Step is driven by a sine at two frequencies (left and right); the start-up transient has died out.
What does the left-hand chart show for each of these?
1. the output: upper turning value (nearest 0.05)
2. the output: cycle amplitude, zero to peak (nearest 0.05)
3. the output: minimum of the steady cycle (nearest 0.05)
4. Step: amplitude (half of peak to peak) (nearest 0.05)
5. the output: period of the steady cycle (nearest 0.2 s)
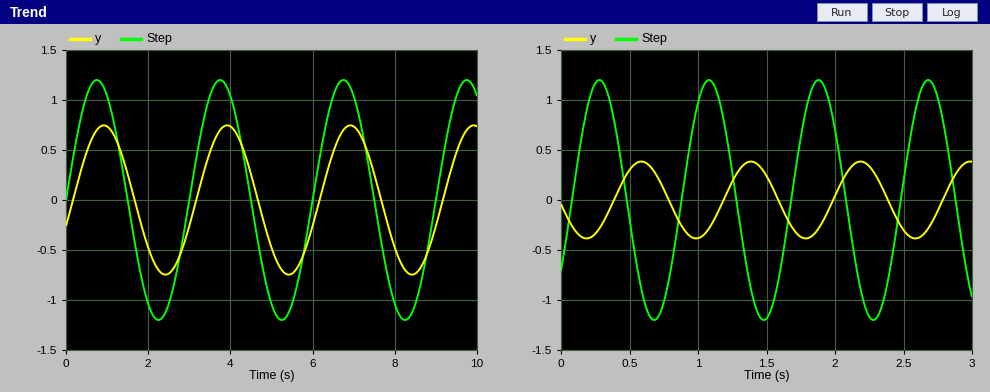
0.75
0.75
-0.75
1.20
3.0 s
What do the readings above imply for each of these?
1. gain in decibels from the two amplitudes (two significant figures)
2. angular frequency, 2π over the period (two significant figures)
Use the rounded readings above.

-4.1 dB
2.1 rad/s
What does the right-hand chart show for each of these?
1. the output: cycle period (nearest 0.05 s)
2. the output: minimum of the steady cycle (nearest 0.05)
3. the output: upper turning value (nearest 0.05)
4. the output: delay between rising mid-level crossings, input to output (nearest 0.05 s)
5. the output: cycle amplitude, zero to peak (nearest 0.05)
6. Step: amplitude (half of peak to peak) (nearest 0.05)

0.80 s
-0.40
0.40
0.30 s
0.40
1.20
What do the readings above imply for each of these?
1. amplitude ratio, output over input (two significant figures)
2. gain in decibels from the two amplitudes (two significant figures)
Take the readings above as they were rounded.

0.33
-9.5 dB
